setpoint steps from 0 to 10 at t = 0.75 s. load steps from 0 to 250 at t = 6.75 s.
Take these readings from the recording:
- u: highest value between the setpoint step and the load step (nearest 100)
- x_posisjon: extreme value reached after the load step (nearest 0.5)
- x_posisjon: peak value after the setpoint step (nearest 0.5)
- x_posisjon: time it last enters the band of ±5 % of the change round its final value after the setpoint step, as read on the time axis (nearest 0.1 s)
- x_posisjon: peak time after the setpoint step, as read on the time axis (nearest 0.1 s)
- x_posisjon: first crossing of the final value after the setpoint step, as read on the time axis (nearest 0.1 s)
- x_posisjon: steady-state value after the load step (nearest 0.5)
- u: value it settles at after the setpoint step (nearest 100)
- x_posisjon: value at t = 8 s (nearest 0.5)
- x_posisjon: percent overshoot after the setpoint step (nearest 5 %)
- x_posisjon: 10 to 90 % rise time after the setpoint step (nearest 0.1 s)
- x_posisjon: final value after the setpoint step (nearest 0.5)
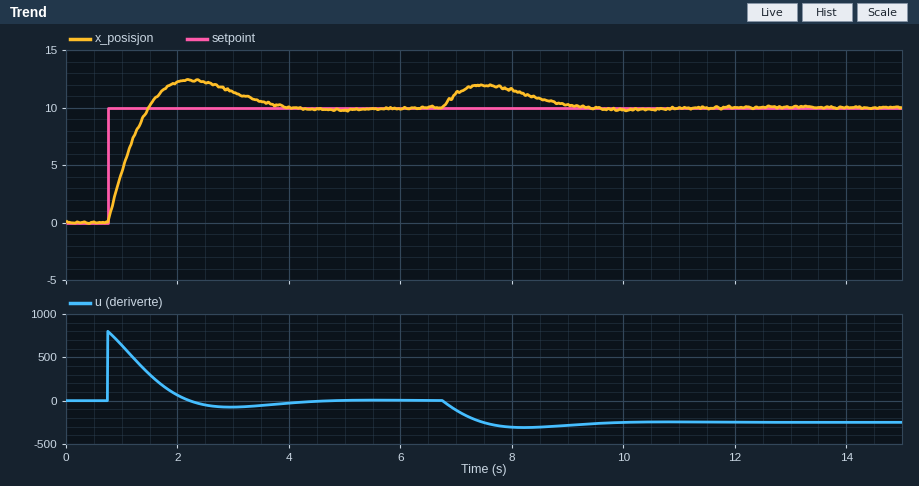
800
12.0
12.5
3.5 s
2.2 s
1.5 s
10.0
0
11.5
25 %
0.6 s
10.0
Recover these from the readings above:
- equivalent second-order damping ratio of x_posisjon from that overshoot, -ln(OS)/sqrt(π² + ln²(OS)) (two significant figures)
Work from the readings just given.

0.40
